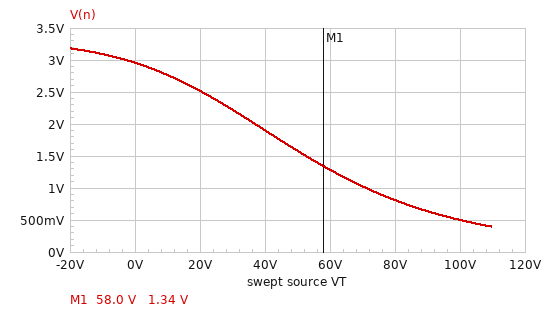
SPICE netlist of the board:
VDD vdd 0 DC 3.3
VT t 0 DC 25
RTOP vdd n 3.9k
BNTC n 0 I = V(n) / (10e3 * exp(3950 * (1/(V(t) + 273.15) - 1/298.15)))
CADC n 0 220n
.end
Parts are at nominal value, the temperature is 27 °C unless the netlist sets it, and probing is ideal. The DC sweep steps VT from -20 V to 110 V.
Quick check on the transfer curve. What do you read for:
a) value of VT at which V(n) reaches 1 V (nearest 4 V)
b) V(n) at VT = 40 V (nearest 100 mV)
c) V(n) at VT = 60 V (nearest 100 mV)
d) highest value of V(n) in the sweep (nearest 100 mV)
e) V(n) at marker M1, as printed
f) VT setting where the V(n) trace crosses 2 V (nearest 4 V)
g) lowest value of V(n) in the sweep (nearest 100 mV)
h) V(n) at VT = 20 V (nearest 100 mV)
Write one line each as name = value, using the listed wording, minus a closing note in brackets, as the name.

value of VT at which V(n) reaches 1 V = 72 V
V(n) at VT = 40 V = 1.9 V
V(n) at VT = 60 V = 1.3 V
highest value of V(n) in the sweep = 3.2 V
V(n) at marker M1, as printed = 1.34 V
VT setting where the V(n) trace crosses 2 V = 36 V
lowest value of V(n) in the sweep = 400 mV
V(n) at VT = 20 V = 2.5 V
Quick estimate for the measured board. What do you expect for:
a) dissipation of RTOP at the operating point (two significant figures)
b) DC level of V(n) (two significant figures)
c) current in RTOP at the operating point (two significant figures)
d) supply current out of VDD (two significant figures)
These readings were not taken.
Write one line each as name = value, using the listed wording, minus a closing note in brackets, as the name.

dissipation of RTOP at the operating point = 220 µW
DC level of V(n) = 2.4 V
current in RTOP at the operating point = 240 µA
supply current out of VDD = 240 µA
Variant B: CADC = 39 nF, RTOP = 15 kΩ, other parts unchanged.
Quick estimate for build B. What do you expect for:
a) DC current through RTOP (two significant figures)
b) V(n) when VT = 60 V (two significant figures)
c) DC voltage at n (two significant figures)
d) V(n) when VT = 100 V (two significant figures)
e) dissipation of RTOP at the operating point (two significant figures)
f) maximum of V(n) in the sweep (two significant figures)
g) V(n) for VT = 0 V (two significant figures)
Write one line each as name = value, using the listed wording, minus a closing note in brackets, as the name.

DC current through RTOP = 130 µA
V(n) when VT = 60 V = 470 mV
DC voltage at n = 1.3 V
V(n) when VT = 100 V = 150 mV
dissipation of RTOP at the operating point = 260 µW
maximum of V(n) in the sweep = 2.9 V
V(n) for VT = 0 V = 2.3 V
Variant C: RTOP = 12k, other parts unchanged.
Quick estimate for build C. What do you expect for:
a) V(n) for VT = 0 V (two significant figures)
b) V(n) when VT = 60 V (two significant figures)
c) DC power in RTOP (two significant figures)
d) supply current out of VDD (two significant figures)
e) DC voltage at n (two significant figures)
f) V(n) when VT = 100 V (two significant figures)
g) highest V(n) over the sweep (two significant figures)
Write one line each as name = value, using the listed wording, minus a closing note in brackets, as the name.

V(n) for VT = 0 V = 2.4 V
V(n) when VT = 60 V = 570 mV
DC power in RTOP = 270 µW
supply current out of VDD = 150 µA
DC voltage at n = 1.5 V
V(n) when VT = 100 V = 180 mV
highest V(n) over the sweep = 3.0 V
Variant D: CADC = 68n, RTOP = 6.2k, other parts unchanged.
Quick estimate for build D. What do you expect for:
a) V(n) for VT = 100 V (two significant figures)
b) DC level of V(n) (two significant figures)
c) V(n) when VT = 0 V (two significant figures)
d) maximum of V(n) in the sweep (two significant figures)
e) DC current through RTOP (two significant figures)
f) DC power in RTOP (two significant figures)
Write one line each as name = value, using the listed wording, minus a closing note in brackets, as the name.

V(n) for VT = 100 V = 330 mV
DC level of V(n) = 2.0 V
V(n) when VT = 0 V = 2.8 V
maximum of V(n) in the sweep = 3.1 V
DC current through RTOP = 200 µA
DC power in RTOP = 260 µW
